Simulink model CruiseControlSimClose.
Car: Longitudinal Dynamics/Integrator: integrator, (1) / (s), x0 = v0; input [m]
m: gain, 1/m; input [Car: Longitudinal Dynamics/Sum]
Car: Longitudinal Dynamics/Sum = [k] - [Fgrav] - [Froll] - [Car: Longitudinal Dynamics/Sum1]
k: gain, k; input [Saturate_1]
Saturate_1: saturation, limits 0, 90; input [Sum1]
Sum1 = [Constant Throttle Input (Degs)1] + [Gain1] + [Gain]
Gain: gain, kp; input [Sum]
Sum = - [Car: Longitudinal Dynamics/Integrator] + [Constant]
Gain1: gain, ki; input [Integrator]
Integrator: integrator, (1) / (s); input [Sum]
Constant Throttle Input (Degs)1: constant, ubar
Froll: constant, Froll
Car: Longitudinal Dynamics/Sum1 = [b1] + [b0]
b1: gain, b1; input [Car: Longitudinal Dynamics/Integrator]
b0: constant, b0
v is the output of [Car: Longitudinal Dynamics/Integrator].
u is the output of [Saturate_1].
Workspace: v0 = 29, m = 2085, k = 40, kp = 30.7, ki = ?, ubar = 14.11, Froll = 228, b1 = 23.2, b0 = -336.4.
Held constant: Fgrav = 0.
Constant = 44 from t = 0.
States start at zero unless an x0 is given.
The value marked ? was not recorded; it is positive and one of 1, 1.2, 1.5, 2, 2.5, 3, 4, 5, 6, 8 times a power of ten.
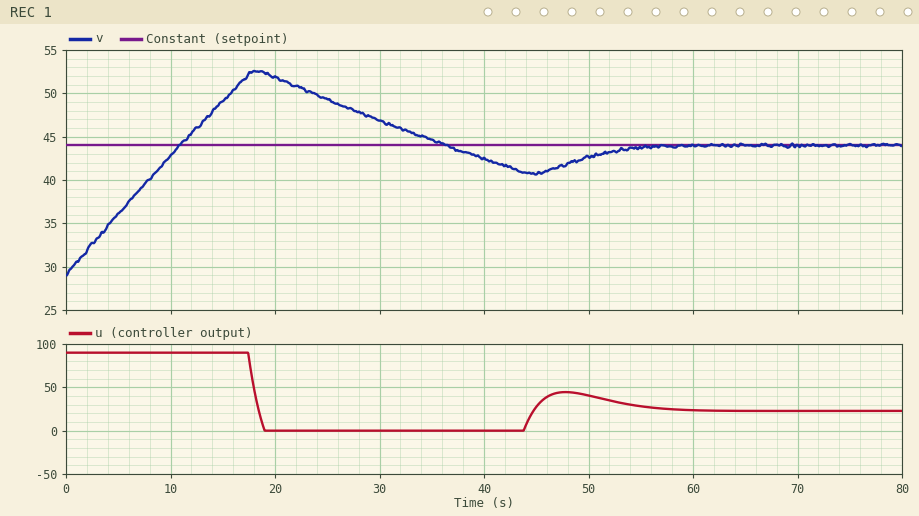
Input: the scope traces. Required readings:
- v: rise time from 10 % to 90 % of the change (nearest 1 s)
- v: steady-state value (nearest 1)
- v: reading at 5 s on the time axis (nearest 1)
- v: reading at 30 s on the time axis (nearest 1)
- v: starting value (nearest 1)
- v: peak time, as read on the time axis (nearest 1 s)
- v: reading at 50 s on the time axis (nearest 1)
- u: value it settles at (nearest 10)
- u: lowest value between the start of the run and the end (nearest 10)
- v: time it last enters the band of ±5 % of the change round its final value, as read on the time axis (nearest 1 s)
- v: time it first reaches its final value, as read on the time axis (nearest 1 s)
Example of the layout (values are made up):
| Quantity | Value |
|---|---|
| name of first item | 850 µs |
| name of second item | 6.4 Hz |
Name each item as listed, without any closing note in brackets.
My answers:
| Quantity | Value |
|---|---|
| v: rise time from 10 % to 90 % of the change | 9 s |
| v: steady-state value | 44 |
| v: reading at 5 s on the time axis | 36 |
| v: reading at 30 s on the time axis | 47 |
| v: starting value | 29 |
| v: peak time, as read on the time axis | 18 s |
| v: reading at 50 s on the time axis | 43 |
| u: value it settles at | 20 |
| u: lowest value between the start of the run and the end | 0 |
| v: time it last enters the band of ±5 % of the change round its final value, as read on the time axis | 52 s |
| v: time it first reaches its final value, as read on the time axis | 11 s |
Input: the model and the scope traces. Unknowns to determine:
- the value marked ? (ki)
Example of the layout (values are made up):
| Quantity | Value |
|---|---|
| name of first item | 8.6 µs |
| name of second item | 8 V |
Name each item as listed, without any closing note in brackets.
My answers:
| Quantity | Value |
|---|---|
| the value marked ? | 6 |
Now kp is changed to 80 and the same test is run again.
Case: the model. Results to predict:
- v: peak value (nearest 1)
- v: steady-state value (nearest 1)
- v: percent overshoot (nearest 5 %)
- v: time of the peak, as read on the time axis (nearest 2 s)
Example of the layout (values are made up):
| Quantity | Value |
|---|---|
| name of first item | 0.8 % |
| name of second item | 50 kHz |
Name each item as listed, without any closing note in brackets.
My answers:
| Quantity | Value |
|---|---|
| v: peak value | 49 |
| v: steady-state value | 44 |
| v: percent overshoot | 35 % |
| v: time of the peak, as read on the time axis | 16 s |
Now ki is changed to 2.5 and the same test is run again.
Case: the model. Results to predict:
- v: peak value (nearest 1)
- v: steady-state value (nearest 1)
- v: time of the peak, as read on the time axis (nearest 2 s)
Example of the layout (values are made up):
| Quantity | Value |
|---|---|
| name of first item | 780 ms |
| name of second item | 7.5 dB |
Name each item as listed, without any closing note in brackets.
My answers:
| Quantity | Value |
|---|---|
| v: peak value | 49 |
| v: steady-state value | 44 |
| v: time of the peak, as read on the time axis | 16 s |
